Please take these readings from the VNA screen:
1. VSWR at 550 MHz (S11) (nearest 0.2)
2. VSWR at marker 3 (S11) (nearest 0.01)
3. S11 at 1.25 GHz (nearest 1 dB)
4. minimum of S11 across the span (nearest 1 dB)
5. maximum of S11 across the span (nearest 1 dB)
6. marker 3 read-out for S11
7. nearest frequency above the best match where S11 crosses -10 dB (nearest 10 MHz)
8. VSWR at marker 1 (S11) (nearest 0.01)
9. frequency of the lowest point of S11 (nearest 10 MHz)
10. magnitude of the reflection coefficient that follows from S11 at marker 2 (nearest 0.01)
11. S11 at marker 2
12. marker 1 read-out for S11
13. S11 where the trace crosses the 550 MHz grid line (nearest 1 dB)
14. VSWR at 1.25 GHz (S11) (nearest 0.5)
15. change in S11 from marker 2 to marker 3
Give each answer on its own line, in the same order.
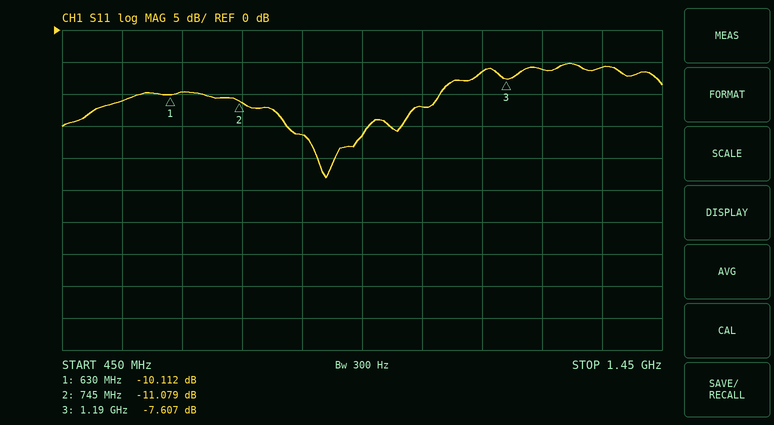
1.8
2.43
-6 dB
-23 dB
-5 dB
-7.607 dB
1.08 GHz
1.91
890 MHz
0.28
-11.079 dB
-10.112 dB
-11 dB
3.0
3.472 dB
